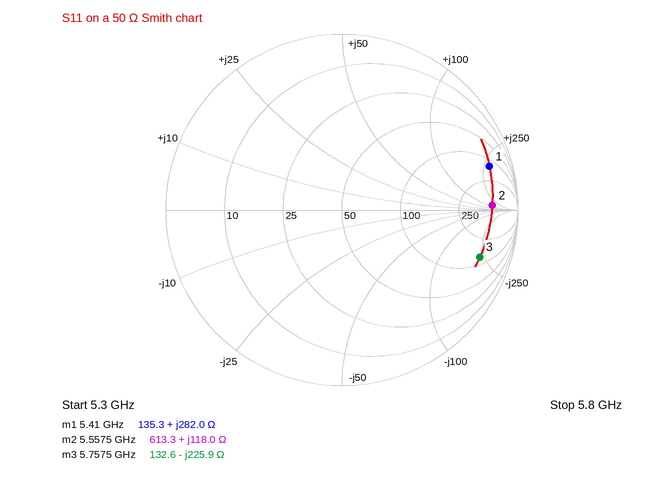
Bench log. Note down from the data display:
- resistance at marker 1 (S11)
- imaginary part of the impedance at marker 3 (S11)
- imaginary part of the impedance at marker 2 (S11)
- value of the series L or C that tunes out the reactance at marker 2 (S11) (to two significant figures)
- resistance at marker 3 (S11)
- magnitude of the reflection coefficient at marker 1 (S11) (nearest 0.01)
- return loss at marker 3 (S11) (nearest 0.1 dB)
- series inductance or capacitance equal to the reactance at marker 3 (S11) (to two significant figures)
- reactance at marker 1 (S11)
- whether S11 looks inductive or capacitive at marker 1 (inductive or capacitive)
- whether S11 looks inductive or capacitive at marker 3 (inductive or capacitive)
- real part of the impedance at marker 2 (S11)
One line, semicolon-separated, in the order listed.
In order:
135.3 Ω; -225.9 Ω; +118.0 Ω; 240 fF; 132.6 Ω; 0.87; 1.6 dB; 120 fF; +282.0 Ω; inductive; capacitive; 613.3 Ω
